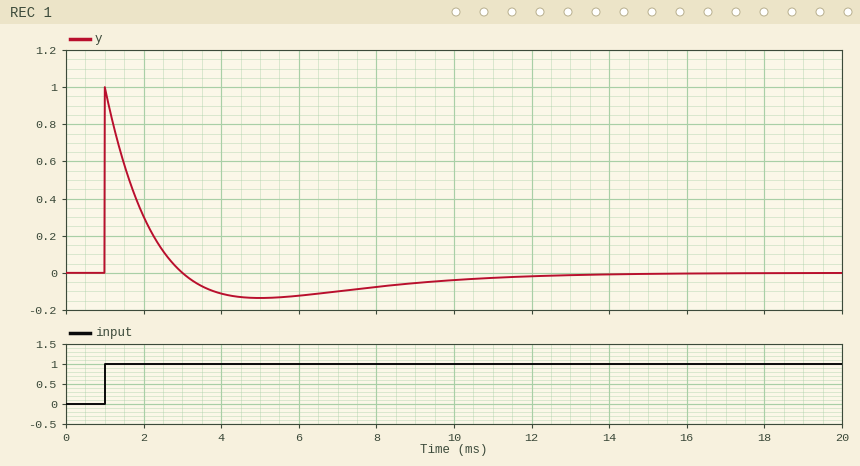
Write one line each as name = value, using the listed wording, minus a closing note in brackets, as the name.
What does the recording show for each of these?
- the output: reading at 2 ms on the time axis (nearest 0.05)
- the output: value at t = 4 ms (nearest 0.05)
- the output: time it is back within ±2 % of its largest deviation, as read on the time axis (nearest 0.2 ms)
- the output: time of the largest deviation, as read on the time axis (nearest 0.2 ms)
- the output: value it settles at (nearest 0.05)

the output: reading at 2 ms on the time axis = 0.30
the output: value at t = 4 ms = -0.10
the output: time it is back within ±2 % of its largest deviation, as read on the time axis = 11.8 ms
the output: time of the largest deviation, as read on the time axis = 1.0 ms
the output: value it settles at = 0.00
